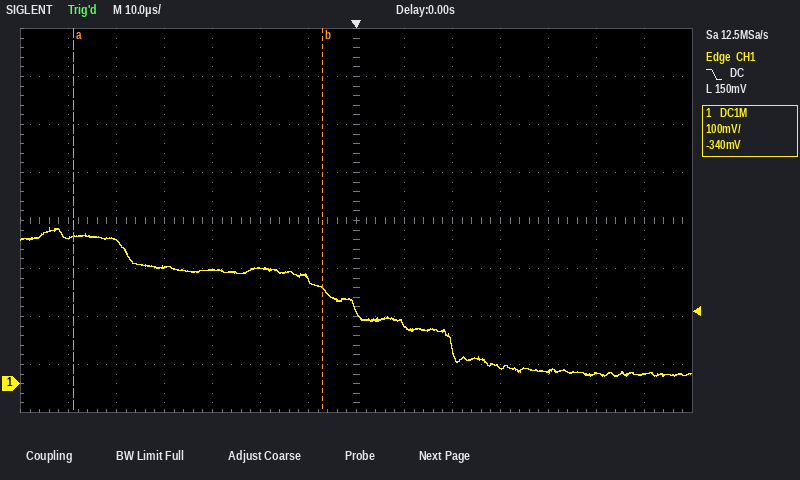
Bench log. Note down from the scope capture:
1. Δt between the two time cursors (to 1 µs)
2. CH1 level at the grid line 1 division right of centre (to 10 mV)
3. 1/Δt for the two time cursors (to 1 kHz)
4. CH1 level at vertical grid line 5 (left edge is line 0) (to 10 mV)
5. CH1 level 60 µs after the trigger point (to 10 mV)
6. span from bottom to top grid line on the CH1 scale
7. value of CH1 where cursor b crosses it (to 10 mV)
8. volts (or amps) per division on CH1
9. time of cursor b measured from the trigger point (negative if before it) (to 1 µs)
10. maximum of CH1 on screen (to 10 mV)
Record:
52 µs
120 mV
19 kHz
240 mV
20 mV
800 mV
200 mV
100 mV
-7 µs
330 mV
